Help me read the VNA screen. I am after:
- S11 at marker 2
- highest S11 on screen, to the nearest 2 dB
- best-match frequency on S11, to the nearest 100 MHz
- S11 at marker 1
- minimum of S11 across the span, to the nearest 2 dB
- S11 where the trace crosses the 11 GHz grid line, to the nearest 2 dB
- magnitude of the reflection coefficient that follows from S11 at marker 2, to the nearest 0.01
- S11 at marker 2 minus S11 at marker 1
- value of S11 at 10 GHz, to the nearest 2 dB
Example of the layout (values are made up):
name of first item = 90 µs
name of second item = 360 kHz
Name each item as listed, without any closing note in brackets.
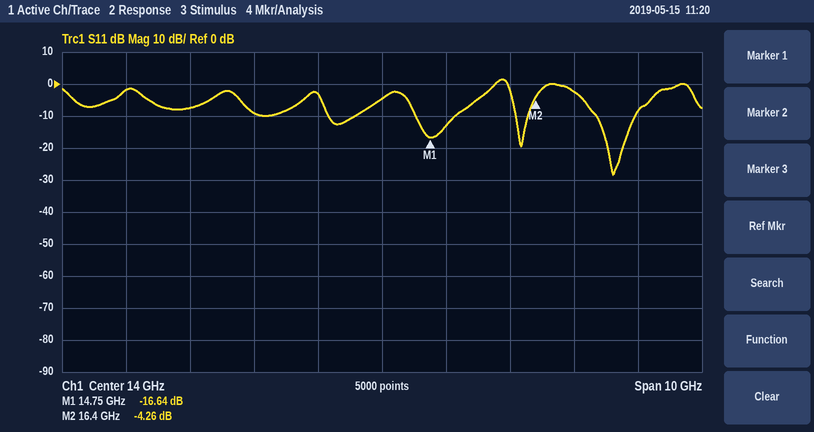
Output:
S11 at marker 2 = -4.26 dB
highest S11 on screen, to the nearest 2 dB = 2 dB
best-match frequency on S11, to the nearest 100 MHz = 17.6 GHz
S11 at marker 1 = -16.64 dB
minimum of S11 across the span, to the nearest 2 dB = -28 dB
S11 where the trace crosses the 11 GHz grid line, to the nearest 2 dB = -8 dB
magnitude of the reflection coefficient that follows from S11 at marker 2, to the nearest 0.01 = 0.61
S11 at marker 2 minus S11 at marker 1 = 12.38 dB
value of S11 at 10 GHz, to the nearest 2 dB = -2 dB
